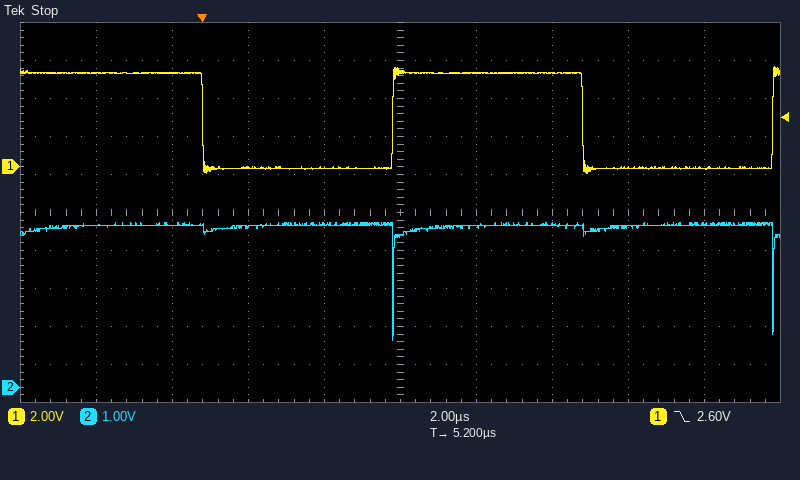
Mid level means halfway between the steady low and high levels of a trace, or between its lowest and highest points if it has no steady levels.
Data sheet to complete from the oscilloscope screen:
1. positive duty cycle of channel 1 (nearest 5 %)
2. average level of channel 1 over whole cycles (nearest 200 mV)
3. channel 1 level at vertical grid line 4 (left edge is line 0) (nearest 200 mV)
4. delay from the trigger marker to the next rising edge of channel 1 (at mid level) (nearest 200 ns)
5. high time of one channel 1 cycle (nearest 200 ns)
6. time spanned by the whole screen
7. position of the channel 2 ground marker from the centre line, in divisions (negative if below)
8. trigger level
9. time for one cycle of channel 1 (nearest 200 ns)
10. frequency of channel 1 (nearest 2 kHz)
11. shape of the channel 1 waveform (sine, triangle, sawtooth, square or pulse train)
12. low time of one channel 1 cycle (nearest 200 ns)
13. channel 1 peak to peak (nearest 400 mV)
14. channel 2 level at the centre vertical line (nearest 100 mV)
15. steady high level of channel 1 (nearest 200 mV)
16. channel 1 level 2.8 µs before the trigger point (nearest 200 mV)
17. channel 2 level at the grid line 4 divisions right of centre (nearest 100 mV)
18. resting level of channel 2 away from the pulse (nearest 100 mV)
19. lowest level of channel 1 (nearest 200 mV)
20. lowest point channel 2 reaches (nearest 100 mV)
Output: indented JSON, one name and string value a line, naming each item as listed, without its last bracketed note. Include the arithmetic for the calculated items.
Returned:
{
  "positive duty cycle of channel 1": "5.0 µs / 10.0 µs ≈ 50 %",
  "average level of channel 1 over whole cycles": "-400 mV + 0.5 × (5.0 V − (-400 mV)) ≈ 2.30 V, so 2.4 V to the nearest 200 mV",
  "channel 1 level at vertical grid line 4 (left edge is line 0)": "0.0 V",
  "delay from the trigger marker to the next rising edge of channel 1 (at mid level)": "5.0 µs",
  "high time of one channel 1 cycle": "5.0 µs",
  "time spanned by the whole screen": "20 µs",
  "position of the channel 2 ground marker from the centre line, in divisions": "-4.6 div",
  "trigger level": "2.60 V",
  "time for one cycle of channel 1": "10.0 µs",
  "frequency of channel 1": "1 / 10.0 µs ≈ 100 kHz",
  "shape of the channel 1 waveform": "square",
  "low time of one channel 1 cycle": "5.0 µs",
  "channel 1 peak to peak": "5.6 V",
  "channel 2 level at the centre vertical line": "4.0 V",
  "steady high level of channel 1": "5.0 V",
  "channel 1 level 2.8 µs before the trigger point": "5.0 V",
  "channel 2 level at the grid line 4 divisions right of centre": "4.3 V",
  "resting level of channel 2 away from the pulse": "4.3 V",
  "lowest level of channel 1": "-400 mV",
  "lowest point channel 2 reaches": "1.2 V"
}
